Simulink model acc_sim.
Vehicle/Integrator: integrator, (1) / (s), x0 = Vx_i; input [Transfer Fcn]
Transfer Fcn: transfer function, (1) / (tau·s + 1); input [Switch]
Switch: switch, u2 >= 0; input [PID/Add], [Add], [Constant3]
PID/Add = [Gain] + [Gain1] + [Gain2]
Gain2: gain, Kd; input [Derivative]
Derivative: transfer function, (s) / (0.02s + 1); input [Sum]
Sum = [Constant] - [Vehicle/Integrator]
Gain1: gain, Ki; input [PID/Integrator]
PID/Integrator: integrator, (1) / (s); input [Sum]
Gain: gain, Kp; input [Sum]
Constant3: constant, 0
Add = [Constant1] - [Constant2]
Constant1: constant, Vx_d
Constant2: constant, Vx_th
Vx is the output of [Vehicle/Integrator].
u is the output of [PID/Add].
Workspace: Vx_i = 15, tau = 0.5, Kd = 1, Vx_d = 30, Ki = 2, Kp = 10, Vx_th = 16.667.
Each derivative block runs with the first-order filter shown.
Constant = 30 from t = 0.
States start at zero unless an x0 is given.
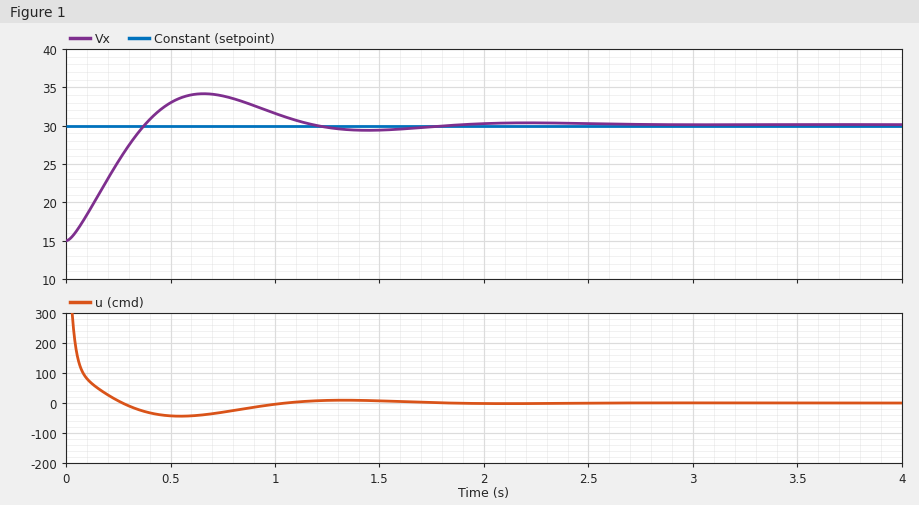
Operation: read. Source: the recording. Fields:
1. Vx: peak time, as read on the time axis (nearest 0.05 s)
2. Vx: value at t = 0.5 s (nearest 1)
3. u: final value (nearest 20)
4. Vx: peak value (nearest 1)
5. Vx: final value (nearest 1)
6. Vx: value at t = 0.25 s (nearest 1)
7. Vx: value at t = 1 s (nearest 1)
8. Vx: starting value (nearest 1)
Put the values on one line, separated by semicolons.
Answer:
0.65 s; 33; 0; 34; 30; 25; 32; 15
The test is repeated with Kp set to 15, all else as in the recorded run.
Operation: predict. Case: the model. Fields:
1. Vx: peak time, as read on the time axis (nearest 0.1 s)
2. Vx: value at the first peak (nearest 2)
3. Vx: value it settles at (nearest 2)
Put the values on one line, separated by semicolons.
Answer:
0.5 s; 36; 30
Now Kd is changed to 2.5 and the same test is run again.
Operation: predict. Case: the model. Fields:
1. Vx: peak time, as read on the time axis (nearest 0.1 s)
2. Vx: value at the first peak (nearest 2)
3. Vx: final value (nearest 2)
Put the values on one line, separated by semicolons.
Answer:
0.6 s; 32; 30
